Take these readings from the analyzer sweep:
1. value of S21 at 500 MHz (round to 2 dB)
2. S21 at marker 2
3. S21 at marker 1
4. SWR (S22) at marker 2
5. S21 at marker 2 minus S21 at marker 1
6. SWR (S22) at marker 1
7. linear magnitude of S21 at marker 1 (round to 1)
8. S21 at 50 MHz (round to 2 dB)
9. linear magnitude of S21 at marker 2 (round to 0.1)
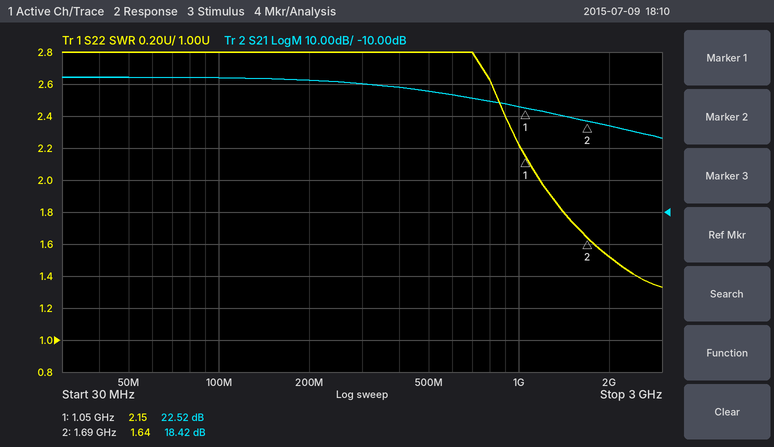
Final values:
28 dB
18.42 dB
22.52 dB
1.64
-4.10 dB
2.15
13
32 dB
8.3
